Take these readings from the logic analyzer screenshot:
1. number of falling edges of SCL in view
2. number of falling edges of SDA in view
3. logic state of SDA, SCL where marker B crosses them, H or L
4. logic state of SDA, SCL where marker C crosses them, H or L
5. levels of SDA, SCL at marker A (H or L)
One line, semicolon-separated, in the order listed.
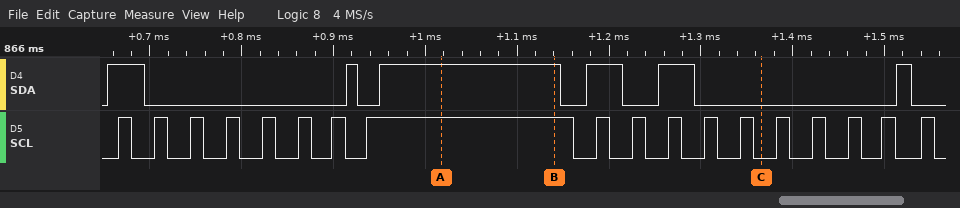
18; 6; SDA=H, SCL=H; SDA=L, SCL=L; SDA=H, SCL=H
